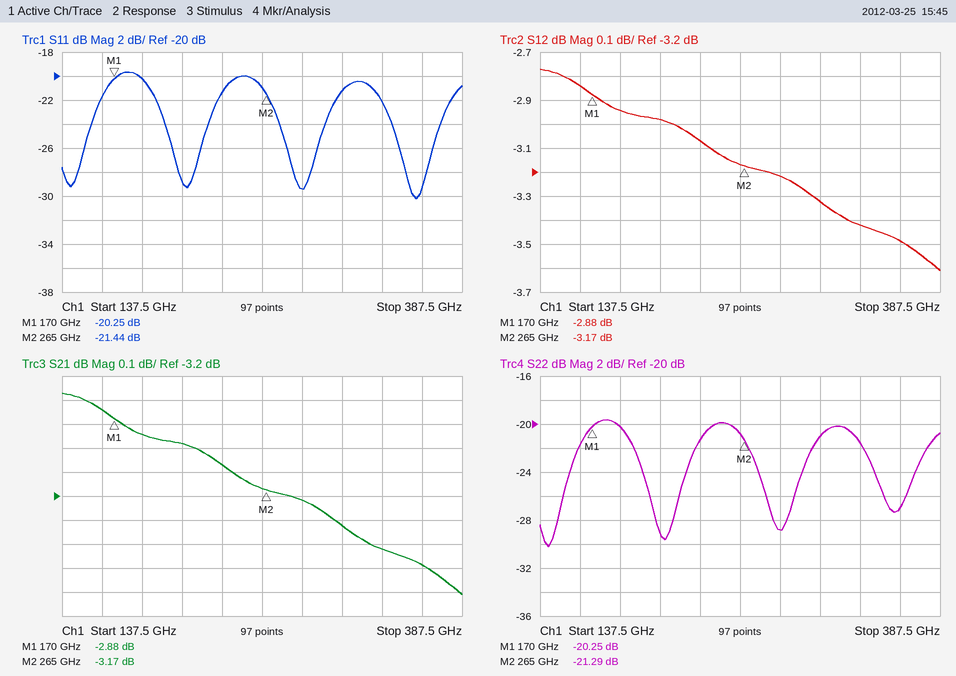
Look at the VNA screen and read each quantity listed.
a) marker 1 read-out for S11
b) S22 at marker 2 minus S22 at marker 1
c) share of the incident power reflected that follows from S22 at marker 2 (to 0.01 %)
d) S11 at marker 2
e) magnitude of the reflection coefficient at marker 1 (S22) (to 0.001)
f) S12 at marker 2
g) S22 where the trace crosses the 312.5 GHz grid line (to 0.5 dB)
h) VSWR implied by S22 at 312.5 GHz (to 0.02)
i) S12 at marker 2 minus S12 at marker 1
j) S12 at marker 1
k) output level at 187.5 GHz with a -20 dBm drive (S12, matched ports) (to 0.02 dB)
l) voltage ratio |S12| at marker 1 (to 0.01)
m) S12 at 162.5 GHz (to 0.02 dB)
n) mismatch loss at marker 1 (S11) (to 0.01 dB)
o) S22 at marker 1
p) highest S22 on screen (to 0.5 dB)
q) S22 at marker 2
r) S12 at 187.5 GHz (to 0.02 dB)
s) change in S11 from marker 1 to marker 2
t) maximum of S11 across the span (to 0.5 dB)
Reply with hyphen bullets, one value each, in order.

- -20.25 dB
- -1.04 dB
- 0.74 %
- -21.44 dB
- 0.097
- -3.17 dB
- -21.0 dB
- 1.20
- -0.29 dB
- -2.88 dB
- -22.94 dBm
- 0.72
- -2.84 dB
- 0.04 dB
- -20.25 dB
- -19.5 dB
- -21.29 dB
- -2.94 dB
- -1.19 dB
- -19.5 dB
